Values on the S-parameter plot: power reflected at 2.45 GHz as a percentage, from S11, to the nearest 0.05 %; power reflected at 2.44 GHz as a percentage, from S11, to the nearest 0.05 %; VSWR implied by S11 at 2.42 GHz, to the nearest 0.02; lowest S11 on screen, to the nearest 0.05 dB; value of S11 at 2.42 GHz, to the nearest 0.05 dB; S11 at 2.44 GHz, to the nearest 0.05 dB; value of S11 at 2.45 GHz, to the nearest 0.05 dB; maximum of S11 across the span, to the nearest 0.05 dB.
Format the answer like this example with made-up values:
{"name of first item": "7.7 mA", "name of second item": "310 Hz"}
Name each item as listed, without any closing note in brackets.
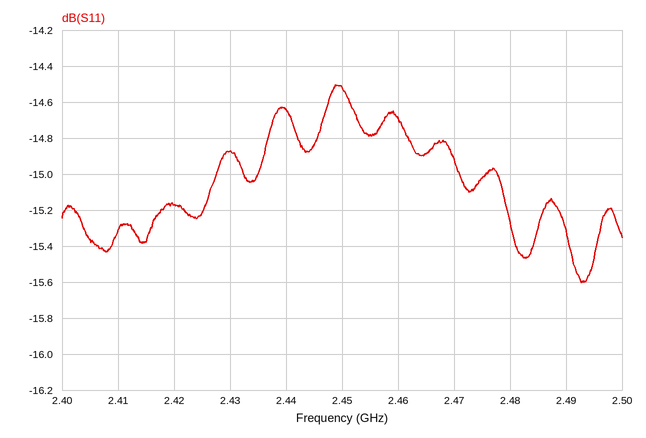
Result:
{"power reflected at 2.45 GHz as a percentage, from S11, to the nearest 0.05 %": "3.55 %", "power reflected at 2.44 GHz as a percentage, from S11, to the nearest 0.05 %": "3.45 %", "VSWR implied by S11 at 2.42 GHz, to the nearest 0.02": "1.42", "lowest S11 on screen, to the nearest 0.05 dB": "-15.60 dB", "value of S11 at 2.42 GHz, to the nearest 0.05 dB": "-15.15 dB", "S11 at 2.44 GHz, to the nearest 0.05 dB": "-14.65 dB", "value of S11 at 2.45 GHz, to the nearest 0.05 dB": "-14.50 dB", "maximum of S11 across the span, to the nearest 0.05 dB": "-14.50 dB"}
